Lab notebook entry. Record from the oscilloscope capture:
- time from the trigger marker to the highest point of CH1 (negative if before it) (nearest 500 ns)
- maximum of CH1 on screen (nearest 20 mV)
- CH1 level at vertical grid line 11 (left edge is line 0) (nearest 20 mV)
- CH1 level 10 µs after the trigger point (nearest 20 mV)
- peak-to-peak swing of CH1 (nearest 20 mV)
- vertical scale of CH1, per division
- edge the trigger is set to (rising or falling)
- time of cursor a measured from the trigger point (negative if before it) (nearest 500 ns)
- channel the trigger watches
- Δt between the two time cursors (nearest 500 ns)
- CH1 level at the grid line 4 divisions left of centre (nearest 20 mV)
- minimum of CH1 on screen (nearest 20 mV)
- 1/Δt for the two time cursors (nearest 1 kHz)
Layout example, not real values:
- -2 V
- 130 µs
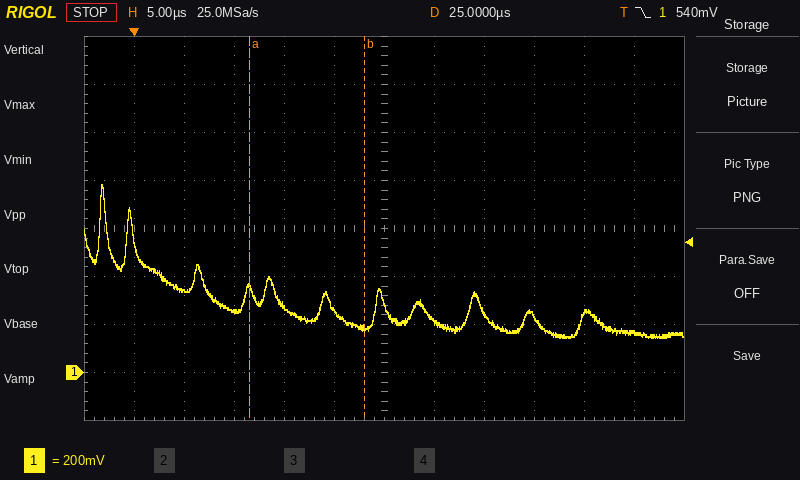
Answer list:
- -3.0 µs
- 780 mV
- 160 mV
- 260 mV
- 640 mV
- 200 mV
- falling
- +11.5 µs
- CH1
- 11.5 µs
- 340 mV
- 140 mV
- 87 kHz
